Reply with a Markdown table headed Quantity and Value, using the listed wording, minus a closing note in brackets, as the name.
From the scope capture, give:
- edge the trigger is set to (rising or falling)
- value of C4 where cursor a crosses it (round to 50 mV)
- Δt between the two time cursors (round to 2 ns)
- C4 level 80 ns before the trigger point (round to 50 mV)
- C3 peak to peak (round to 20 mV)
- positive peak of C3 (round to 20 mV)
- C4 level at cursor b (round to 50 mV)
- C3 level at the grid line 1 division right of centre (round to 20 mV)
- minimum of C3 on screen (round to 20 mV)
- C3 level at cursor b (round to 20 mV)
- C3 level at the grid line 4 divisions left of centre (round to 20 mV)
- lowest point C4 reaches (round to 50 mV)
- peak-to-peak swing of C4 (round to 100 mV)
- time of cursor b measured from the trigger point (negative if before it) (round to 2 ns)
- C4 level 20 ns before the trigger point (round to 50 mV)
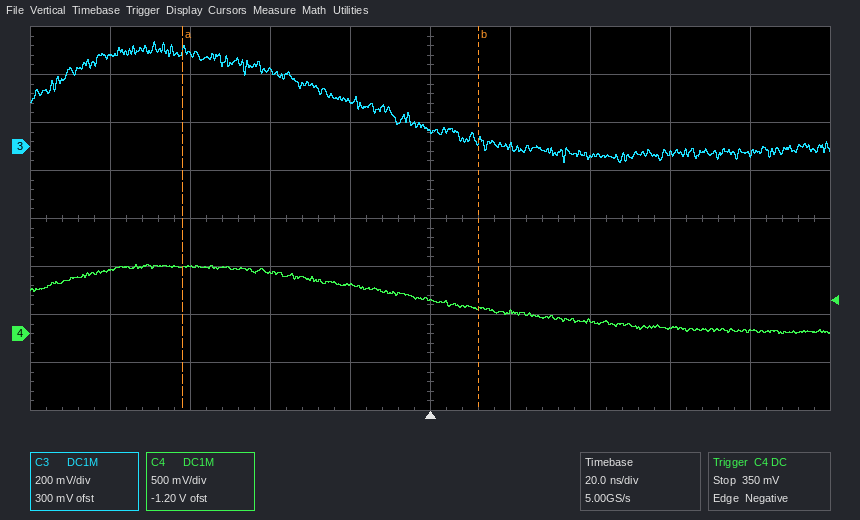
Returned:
| Quantity | Value |
|---|---|
| edge the trigger is set to | falling |
| value of C4 where cursor a crosses it | 700 mV |
| Δt between the two time cursors | 74 ns |
| C4 level 80 ns before the trigger point | 650 mV |
| C3 peak to peak | 500 mV |
| positive peak of C3 | 440 mV |
| C4 level at cursor b | 250 mV |
| C3 level at the grid line 1 division right of centre | 0 mV |
| minimum of C3 on screen | -60 mV |
| C3 level at cursor b | 20 mV |
| C3 level at the grid line 4 divisions left of centre | 380 mV |
| lowest point C4 reaches | 0 mV |
| peak-to-peak swing of C4 | 700 mV |
| time of cursor b measured from the trigger point (negative if before it) | +12 ns |
| C4 level 20 ns before the trigger point | 500 mV |
